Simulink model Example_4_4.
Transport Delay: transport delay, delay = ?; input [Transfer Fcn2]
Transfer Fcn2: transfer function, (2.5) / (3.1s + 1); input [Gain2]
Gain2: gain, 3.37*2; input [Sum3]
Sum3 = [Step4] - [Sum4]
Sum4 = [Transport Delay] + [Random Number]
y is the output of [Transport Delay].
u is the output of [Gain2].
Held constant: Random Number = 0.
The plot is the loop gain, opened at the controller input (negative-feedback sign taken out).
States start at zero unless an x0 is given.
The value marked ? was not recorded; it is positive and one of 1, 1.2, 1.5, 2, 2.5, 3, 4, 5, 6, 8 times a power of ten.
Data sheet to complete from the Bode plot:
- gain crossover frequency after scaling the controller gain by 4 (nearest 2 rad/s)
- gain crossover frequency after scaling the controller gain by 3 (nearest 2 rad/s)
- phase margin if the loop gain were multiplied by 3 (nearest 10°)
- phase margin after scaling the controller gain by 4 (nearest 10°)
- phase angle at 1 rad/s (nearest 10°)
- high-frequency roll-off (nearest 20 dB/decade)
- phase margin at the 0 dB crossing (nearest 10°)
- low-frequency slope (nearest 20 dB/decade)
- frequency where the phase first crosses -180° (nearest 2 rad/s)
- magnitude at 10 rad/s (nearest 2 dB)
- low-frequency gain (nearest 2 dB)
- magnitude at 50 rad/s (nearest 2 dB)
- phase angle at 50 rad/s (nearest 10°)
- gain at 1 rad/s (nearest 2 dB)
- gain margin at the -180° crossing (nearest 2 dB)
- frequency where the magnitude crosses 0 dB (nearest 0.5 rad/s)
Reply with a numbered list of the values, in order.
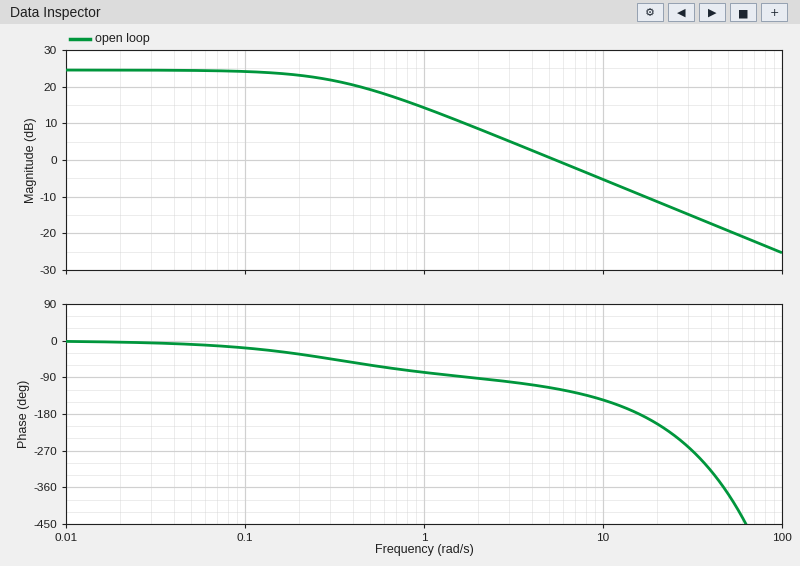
1. 22 rad/s
2. 16 rad/s
3. 0°
4. -30°
5. -80°
6. -20 dB/decade
7. 60°
8. 0 dB/decade
9. 16 rad/s
10. -6 dB
11. 24 dB
12. -20 dB
13. -380°
14. 14 dB
15. 10 dB
16. 5.5 rad/s
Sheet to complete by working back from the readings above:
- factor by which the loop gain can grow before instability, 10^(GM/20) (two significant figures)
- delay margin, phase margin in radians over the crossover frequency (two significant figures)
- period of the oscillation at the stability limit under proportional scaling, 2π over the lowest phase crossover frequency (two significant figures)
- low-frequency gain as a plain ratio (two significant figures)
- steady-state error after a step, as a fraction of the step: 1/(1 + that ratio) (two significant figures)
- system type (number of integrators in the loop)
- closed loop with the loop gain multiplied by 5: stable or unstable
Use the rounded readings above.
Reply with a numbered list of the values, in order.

1. 3.2
2. 0.19 s
3. 0.39 s
4. 16
5. 0.059
6. 0
7. unstable
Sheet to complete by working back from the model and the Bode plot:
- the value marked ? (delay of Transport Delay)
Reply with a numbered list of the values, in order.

1. 0.1
